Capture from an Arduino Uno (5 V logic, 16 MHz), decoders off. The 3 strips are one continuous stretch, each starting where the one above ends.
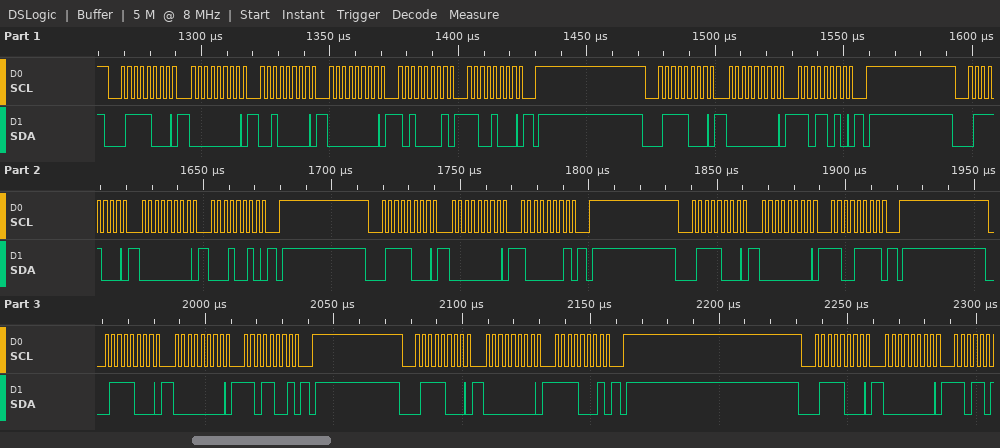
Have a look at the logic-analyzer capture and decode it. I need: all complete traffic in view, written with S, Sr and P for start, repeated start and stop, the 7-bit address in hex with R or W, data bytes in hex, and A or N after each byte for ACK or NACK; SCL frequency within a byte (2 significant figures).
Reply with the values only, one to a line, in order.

S 3CW A 00 A 20 A 00 A A1 A C8 A P S 3CW A 00 A DA A P S 3CW A 00 A 12 A P S 3CW A 00 A 81 A P S 3CW A 00 A CF A P S 3CW A 00 A D9 A P S 3CW A 00 A F1 A P S 3CW A 00 A
400 kHz
